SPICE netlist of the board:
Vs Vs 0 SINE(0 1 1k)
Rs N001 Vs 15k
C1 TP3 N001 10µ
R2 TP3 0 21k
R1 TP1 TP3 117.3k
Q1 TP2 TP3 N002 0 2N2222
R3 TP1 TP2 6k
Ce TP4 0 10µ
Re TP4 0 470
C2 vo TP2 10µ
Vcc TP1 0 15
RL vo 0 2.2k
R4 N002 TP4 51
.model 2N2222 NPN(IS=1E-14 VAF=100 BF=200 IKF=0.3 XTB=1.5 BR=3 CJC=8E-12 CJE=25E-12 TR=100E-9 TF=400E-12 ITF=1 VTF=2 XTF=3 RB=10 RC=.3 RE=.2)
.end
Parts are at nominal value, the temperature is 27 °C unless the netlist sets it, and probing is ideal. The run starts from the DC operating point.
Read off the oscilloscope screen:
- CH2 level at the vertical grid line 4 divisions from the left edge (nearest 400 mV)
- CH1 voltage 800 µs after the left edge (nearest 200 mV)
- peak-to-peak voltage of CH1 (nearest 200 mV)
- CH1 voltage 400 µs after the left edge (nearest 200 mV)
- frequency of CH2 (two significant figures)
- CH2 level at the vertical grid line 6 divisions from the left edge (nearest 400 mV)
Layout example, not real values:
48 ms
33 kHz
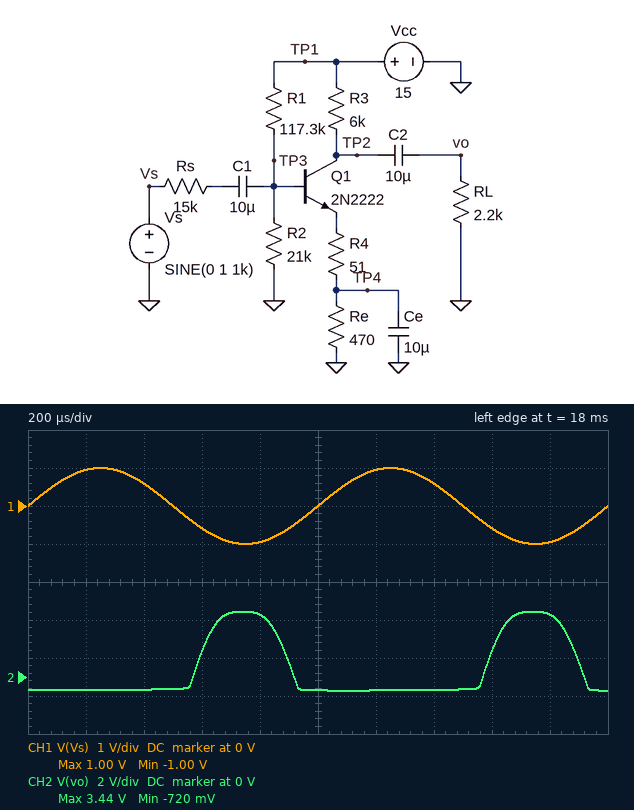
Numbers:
3.2 V
-1.0 V
2.0 V
600 mV
1.0 kHz
-800 mV
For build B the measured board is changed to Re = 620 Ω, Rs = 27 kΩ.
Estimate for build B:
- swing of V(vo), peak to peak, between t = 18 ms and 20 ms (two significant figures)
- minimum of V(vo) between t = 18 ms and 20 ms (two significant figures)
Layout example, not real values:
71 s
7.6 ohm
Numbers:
4.4 V
-1.3 V
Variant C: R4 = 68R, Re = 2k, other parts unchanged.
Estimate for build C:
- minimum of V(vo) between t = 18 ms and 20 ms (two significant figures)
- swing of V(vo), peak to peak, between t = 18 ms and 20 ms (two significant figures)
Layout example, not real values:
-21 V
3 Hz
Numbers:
-3.9 V
5.2 V
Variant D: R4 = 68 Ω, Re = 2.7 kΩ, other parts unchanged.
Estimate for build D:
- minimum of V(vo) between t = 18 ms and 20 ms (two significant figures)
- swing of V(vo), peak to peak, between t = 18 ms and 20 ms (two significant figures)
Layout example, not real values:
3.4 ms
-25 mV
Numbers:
-3.4 V
4.4 V
